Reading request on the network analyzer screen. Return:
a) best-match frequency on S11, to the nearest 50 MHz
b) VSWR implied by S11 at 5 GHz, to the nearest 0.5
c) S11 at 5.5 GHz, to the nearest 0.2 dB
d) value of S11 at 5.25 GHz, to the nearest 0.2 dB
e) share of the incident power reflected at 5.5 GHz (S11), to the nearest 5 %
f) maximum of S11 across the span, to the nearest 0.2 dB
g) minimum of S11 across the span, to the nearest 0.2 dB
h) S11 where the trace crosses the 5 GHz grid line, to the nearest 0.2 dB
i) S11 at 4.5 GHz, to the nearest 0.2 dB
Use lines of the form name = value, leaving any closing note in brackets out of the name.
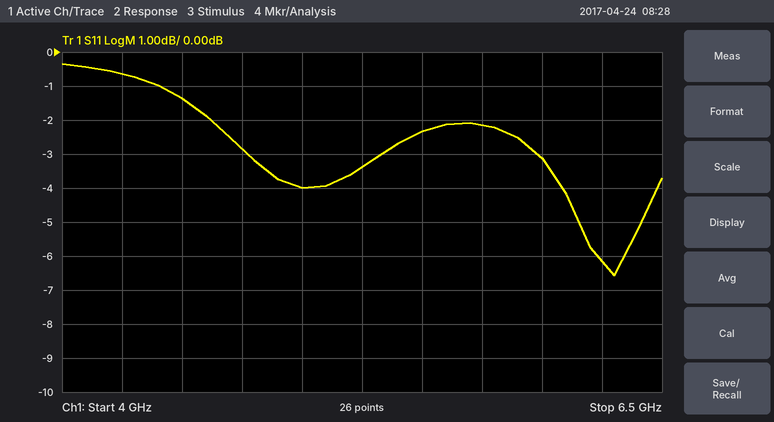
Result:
best-match frequency on S11, to the nearest 50 MHz = 6.30 GHz
VSWR implied by S11 at 5 GHz, to the nearest 0.5 = 4.5
S11 at 5.5 GHz, to the nearest 0.2 dB = -2.4 dB
value of S11 at 5.25 GHz, to the nearest 0.2 dB = -3.4 dB
share of the incident power reflected at 5.5 GHz (S11), to the nearest 5 % = 60 %
maximum of S11 across the span, to the nearest 0.2 dB = -0.4 dB
minimum of S11 across the span, to the nearest 0.2 dB = -6.6 dB
S11 where the trace crosses the 5 GHz grid line, to the nearest 0.2 dB = -4.0 dB
S11 at 4.5 GHz, to the nearest 0.2 dB = -1.4 dB
